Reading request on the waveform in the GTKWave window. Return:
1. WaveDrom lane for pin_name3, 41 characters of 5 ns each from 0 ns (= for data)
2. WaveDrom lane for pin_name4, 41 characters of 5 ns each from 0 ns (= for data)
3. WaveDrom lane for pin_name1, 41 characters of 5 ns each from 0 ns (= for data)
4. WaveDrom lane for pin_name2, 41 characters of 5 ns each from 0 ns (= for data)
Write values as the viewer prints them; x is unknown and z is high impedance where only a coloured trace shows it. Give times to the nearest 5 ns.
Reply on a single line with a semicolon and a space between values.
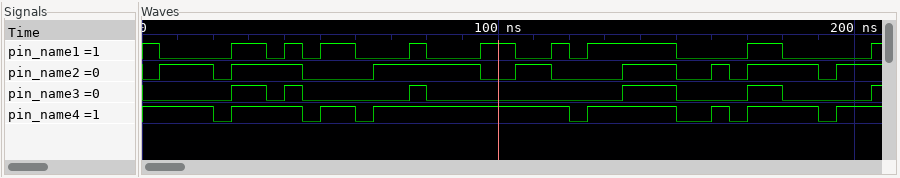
{name: 'pin_name3', wave: '0....1.010.....10..........1..0...1.0....'}; {name: 'pin_name4', wave: '1...01...01.01..........01....0.101...01.'}; {name: 'pin_name1', wave: '10...1.0101.0..10..1.0.101....0...1.0....'}; {name: 'pin_name2', wave: '01..01...0...1.....0.1.0...1..0.101...01.'}
